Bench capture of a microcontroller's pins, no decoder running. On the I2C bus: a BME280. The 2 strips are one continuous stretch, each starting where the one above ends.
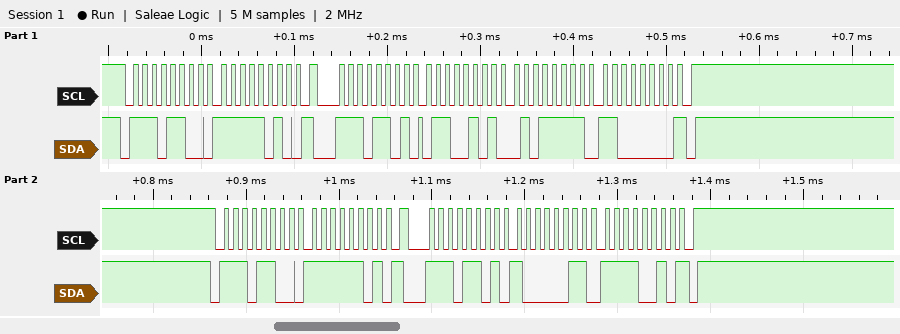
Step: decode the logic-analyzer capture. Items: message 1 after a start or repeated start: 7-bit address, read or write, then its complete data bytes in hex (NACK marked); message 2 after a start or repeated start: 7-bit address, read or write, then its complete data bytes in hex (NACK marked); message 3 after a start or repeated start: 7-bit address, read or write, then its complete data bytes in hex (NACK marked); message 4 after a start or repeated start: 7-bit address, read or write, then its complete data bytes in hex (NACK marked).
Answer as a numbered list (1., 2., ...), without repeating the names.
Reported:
1. 0x76 write: FA
2. 0x76 read: 65 5F C0 NACK
3. 0x76 write: FD
4. 0x76 read: 83 F2 NACK
